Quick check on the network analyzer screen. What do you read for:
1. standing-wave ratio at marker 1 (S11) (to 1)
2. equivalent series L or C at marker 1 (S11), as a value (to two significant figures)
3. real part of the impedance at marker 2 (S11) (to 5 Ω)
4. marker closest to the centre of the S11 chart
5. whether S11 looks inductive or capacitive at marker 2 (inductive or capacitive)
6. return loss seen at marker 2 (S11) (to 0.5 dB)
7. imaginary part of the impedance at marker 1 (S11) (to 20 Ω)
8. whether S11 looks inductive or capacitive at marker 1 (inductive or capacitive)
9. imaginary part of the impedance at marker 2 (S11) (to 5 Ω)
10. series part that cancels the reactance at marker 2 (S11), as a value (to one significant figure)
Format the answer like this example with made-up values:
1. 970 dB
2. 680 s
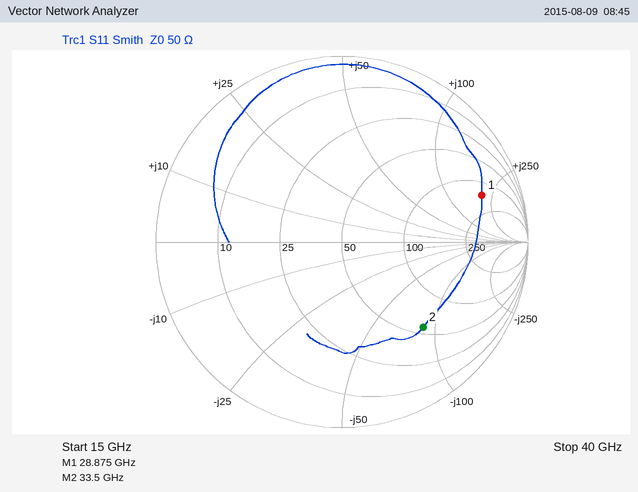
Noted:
1. 9
2. 1.1 nH
3. 55 Ω
4. marker 2
5. capacitive
6. 4.0 dB
7. +200 Ω
8. inductive
9. -85 Ω
10. 400 pH
